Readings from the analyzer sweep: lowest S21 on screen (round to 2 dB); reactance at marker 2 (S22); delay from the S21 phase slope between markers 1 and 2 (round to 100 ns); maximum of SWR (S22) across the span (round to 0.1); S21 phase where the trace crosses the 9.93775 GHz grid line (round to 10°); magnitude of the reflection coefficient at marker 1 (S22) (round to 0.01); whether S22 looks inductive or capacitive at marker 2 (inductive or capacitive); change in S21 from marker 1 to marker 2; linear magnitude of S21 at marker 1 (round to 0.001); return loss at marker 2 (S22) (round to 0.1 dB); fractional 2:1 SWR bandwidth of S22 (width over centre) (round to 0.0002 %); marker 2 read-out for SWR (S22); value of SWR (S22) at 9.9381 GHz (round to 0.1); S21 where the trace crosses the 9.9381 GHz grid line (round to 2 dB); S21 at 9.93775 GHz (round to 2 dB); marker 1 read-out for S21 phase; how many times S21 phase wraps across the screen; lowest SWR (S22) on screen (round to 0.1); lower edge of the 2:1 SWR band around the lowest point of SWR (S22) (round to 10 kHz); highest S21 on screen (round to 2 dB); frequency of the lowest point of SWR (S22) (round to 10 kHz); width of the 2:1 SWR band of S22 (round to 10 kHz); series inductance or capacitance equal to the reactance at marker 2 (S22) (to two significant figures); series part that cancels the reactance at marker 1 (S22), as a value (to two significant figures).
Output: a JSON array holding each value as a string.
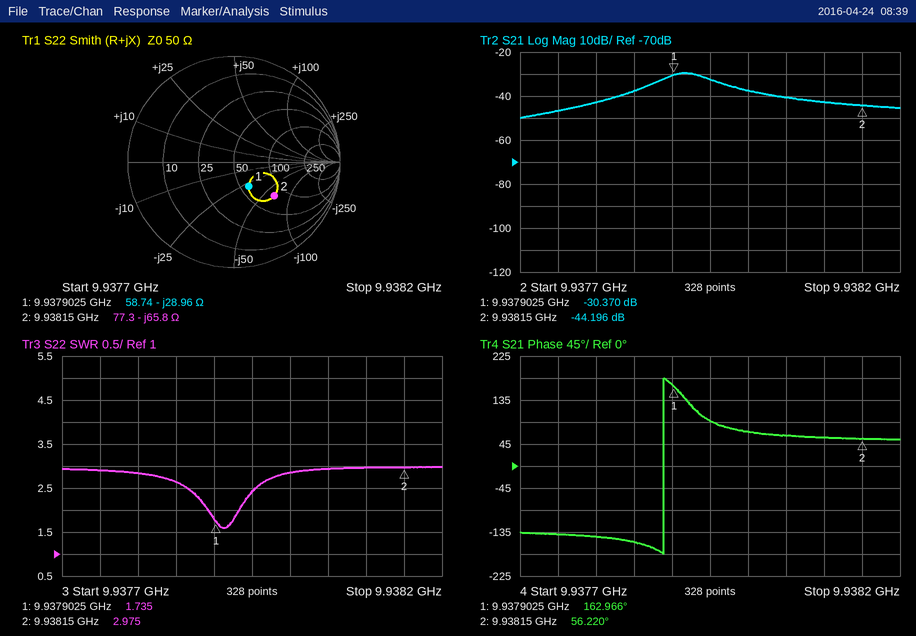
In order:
["-50 dB", "-65.8 Ω", "1.2 µs", "3.0", "-140°", "0.27", "capacitive", "-13.826 dB", "0.030", "6.1 dB", "0.0004 %", "2.975", "3.0", "-42 dB", "-46 dB", "162.966°", "1", "1.6", "9.93789 GHz", "-30 dB", "9.93791 GHz", "40 kHz", "240 fF", "460 pH"]
